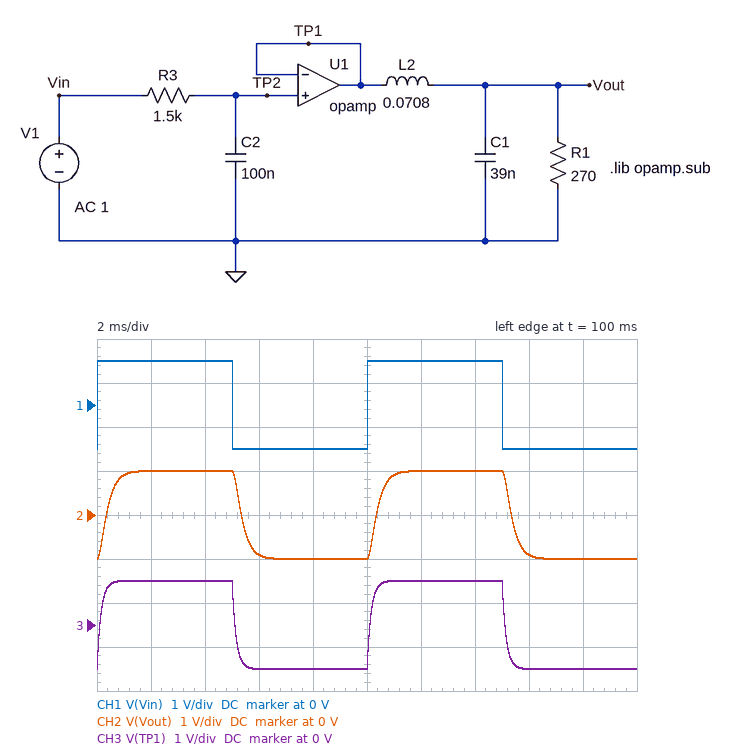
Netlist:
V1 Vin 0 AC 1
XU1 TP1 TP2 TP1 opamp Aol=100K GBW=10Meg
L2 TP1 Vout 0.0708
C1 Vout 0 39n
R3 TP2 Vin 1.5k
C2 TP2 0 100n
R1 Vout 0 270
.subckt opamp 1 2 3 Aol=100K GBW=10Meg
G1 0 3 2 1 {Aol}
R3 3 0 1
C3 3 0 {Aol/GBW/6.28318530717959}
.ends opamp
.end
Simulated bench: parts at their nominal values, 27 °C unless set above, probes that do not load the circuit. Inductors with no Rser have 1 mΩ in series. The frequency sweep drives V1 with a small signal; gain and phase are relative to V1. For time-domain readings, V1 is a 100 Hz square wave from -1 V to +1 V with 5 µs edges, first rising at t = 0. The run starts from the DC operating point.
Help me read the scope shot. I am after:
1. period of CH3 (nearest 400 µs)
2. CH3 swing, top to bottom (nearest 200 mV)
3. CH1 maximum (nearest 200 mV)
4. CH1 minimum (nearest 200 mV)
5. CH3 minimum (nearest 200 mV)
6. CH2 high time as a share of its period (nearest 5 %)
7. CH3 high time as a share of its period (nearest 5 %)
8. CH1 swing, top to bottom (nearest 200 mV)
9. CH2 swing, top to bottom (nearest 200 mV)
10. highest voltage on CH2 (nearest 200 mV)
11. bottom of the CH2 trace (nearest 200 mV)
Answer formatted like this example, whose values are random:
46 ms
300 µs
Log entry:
10.0 ms
2.0 V
1.0 V
-1.0 V
-1.0 V
50 %
50 %
2.0 V
2.0 V
1.0 V
-1.0 V
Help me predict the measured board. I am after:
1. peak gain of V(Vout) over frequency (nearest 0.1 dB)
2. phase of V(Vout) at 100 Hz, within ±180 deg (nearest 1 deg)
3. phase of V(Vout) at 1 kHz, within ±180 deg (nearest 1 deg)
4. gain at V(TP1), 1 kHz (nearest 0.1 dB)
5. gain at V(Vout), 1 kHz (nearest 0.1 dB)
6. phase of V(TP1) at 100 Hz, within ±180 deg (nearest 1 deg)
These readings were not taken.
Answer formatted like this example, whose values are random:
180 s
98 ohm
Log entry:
0 dB
-15 deg
-105 deg
-2.8 dB
-8.2 dB
-5 deg
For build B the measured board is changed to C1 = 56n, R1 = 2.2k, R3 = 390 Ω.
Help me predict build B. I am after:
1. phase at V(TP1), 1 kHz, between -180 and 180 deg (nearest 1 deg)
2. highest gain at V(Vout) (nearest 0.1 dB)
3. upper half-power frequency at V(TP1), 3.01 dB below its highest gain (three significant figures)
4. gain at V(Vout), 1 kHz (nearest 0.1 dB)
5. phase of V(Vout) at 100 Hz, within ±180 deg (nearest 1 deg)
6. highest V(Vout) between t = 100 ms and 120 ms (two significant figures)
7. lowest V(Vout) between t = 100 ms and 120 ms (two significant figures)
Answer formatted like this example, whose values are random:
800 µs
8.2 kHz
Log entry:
-14 deg
4.9 dB
4.08 kHz
1.0 dB
-3 deg
1.7 V
-1.7 V
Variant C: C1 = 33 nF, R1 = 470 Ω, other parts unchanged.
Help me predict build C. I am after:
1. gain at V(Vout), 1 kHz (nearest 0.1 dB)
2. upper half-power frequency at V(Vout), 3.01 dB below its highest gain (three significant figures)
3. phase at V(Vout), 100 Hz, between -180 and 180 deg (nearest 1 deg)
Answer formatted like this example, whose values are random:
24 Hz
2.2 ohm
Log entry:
-5.1 dB
719 Hz
-11 deg
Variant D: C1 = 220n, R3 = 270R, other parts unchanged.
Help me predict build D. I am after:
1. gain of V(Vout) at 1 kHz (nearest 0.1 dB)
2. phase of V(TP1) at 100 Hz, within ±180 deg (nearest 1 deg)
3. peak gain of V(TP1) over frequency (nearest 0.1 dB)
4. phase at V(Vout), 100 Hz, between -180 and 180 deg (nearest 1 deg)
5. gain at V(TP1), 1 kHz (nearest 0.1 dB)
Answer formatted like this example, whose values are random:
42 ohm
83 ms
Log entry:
-4.7 dB
-1 deg
0 dB
-10 deg
-0.1 dB
